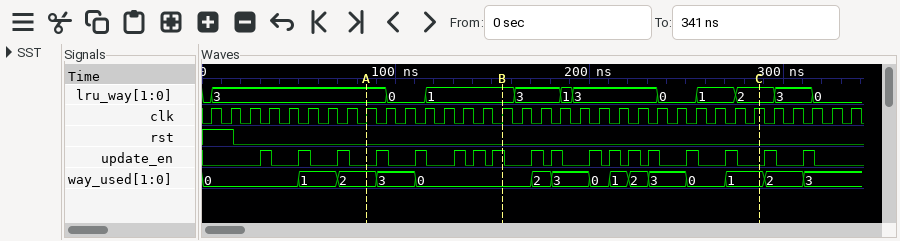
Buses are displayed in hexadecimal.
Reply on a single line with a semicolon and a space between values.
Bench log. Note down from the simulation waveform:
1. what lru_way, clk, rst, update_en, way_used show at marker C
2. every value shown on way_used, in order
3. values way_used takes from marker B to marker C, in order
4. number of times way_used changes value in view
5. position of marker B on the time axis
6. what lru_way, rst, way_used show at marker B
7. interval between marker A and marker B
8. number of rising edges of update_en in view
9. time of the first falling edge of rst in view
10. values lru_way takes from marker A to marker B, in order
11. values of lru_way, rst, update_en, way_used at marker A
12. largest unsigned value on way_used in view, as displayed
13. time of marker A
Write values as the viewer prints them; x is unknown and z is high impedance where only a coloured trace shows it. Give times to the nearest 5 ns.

lru_way=2, clk=1, rst=0, update_en=0, way_used=1; 0, 1, 2, 3, 0, 2, 3, 0, 1, 2, 3, 0, 1, 2, 3; 0, 2, 3, 0, 1, 2, 3, 0, 1; 14; 155 ns; lru_way=1, rst=0, way_used=0; 70 ns; 18; 15 ns; 3, 0, 1; lru_way=3, rst=0, update_en=0, way_used=2; 3; 85 ns
